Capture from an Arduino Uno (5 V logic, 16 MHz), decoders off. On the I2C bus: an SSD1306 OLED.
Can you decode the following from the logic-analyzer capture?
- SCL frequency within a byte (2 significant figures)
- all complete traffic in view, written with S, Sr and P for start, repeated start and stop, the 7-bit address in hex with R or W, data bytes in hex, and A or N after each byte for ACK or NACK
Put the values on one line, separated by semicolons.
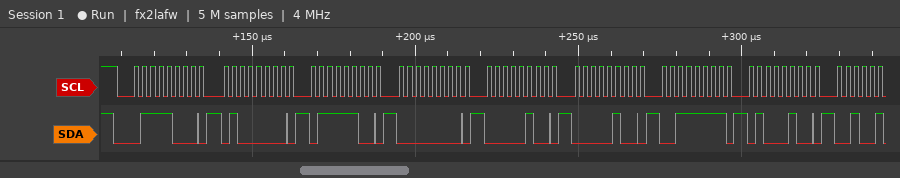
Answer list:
400 kHz; S 3CW A 40 A 7C A 00 A 04 A 04 A 3F A 44 A
